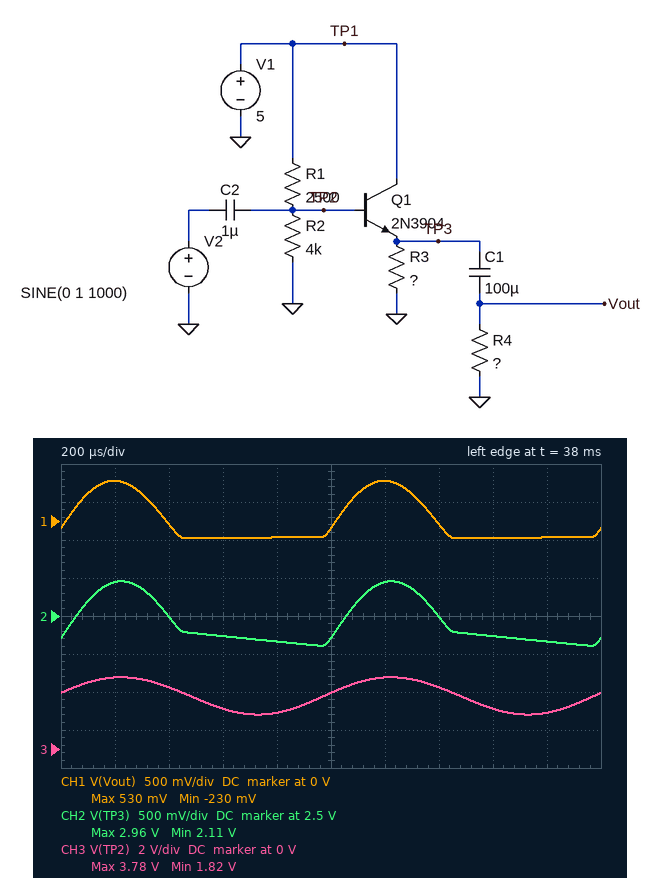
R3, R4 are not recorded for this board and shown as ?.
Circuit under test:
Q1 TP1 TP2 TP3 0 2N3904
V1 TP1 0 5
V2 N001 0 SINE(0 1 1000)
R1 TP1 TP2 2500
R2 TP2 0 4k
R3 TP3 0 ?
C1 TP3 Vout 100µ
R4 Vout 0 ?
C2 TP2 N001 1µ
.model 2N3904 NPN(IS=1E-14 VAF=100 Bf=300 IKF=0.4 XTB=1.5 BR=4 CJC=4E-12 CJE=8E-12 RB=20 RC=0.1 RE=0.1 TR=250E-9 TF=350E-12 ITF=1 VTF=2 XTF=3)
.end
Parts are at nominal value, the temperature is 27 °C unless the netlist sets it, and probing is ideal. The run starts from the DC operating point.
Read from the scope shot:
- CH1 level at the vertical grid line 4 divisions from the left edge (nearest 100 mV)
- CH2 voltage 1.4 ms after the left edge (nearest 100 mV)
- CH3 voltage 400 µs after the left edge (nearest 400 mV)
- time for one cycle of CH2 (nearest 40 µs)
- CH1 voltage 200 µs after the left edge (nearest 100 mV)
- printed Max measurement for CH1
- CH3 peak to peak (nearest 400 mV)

-200 mV
2.5 V
3.2 V
1.00 ms
500 mV
530 mV
2.0 V
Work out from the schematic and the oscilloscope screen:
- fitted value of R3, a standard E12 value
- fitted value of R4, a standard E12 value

56 Ω
5.6 Ω
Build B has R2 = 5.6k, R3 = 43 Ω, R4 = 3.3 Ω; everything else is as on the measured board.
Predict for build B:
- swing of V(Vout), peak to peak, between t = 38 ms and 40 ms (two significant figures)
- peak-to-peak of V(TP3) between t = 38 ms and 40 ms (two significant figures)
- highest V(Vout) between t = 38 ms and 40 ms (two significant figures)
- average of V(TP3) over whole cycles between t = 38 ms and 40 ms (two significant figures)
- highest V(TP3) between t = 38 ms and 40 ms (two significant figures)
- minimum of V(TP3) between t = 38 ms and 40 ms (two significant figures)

660 mV
810 mV
470 mV
2.6 V
3.1 V
2.3 V
